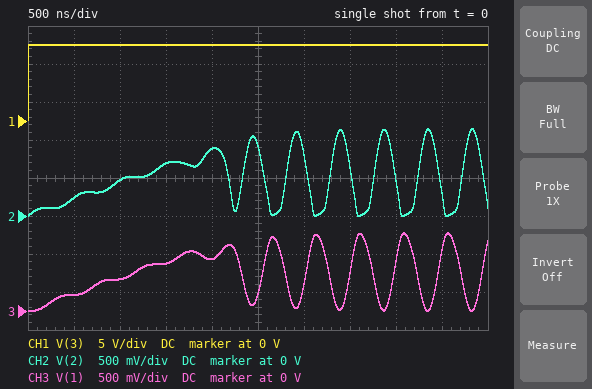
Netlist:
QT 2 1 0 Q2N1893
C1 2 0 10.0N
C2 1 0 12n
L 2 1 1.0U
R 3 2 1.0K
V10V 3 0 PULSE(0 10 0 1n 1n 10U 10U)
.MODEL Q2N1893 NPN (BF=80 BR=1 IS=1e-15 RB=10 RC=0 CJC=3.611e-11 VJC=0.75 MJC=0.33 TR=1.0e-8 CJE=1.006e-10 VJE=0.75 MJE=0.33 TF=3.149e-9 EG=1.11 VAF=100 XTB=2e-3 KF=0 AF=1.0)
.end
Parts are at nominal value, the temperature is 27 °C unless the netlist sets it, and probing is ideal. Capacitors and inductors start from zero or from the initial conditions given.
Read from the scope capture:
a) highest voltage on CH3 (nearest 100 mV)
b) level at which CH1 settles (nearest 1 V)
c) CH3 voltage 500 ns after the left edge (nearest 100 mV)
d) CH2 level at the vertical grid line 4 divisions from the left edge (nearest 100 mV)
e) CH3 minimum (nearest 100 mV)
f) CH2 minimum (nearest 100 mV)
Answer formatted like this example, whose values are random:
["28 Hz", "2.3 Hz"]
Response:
["1.0 V", "10 V", "200 mV", "900 mV", "0 V", "0 V"]
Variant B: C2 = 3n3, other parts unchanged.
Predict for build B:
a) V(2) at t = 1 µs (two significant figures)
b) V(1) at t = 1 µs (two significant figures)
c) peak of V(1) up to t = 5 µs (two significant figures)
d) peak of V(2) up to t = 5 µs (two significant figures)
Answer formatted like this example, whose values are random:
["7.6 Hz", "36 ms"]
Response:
["720 mV", "690 mV", "980 mV", "800 mV"]
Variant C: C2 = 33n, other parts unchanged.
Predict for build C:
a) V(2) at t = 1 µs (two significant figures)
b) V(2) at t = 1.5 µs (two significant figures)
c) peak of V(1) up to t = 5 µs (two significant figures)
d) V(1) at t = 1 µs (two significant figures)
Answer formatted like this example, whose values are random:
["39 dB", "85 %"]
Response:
["170 mV", "280 mV", "920 mV", "250 mV"]
